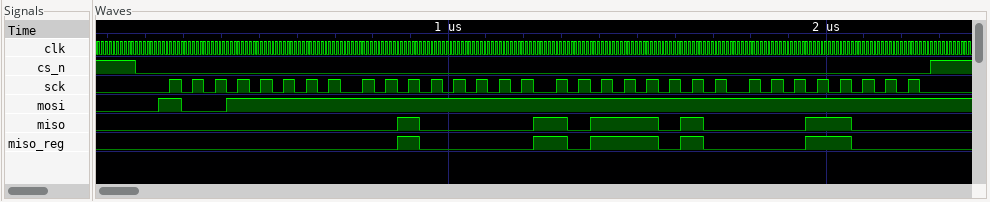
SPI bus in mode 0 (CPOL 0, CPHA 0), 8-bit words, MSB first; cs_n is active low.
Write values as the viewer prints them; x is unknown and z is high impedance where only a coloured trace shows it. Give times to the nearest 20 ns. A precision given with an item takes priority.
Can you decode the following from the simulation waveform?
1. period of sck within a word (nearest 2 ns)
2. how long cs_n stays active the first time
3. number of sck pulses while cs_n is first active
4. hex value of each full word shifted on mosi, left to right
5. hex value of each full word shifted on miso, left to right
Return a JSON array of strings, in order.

["60 ns", "2100 ns", "32", "9F, FF, FF, FF", "00, 20, BA, 18"]
